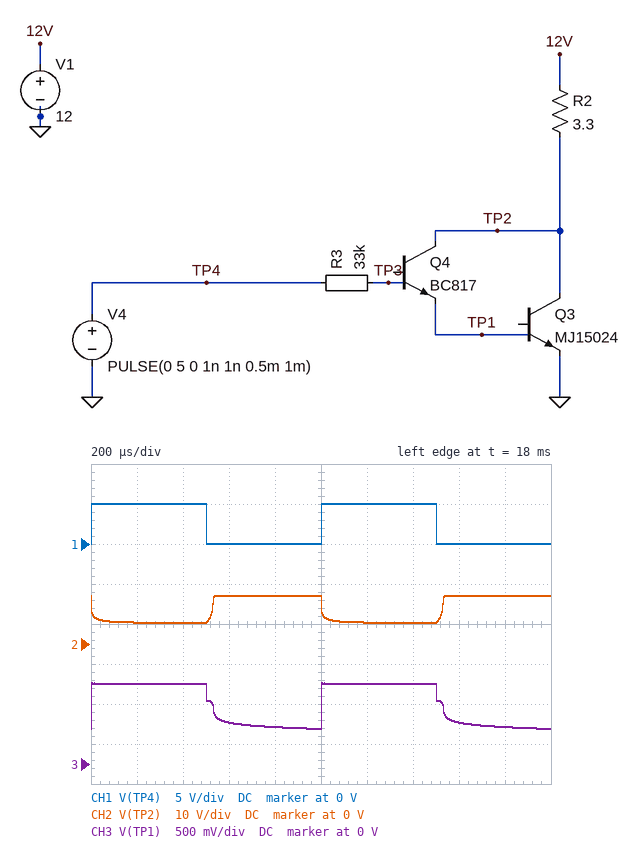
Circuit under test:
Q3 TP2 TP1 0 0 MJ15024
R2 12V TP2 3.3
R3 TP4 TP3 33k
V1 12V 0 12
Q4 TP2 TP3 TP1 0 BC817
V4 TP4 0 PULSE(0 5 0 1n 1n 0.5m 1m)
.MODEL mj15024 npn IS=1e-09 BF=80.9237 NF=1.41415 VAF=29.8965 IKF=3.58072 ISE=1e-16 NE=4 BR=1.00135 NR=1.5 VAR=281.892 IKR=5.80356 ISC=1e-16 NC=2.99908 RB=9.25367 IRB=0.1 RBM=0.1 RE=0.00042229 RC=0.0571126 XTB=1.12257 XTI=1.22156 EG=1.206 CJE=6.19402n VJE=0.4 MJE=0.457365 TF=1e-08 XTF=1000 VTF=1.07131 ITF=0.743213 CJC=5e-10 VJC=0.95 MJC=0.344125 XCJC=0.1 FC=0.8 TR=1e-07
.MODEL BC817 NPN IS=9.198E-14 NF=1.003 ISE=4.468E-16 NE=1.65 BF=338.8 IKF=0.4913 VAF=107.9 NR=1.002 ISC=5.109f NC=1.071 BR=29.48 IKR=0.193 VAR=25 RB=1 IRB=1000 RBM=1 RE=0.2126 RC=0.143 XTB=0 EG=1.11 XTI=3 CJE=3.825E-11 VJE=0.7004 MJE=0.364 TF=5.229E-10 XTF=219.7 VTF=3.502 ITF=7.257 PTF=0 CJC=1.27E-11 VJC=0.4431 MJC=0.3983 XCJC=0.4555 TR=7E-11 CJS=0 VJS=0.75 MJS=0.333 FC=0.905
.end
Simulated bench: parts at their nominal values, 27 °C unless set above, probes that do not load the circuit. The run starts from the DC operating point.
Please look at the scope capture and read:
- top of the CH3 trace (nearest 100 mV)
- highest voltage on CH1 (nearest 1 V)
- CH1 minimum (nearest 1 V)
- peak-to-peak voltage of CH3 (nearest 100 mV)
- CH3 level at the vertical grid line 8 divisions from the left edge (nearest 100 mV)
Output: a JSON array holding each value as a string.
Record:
["1.0 V", "5 V", "0 V", "600 mV", "500 mV"]
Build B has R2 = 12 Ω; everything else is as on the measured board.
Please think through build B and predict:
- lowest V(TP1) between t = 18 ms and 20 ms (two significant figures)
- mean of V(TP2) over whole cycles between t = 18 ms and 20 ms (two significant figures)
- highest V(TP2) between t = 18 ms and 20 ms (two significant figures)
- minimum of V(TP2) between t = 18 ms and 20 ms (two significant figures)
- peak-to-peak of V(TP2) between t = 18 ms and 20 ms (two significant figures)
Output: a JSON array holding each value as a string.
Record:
["470 mV", "4.1 V", "12 V", "940 mV", "11 V"]
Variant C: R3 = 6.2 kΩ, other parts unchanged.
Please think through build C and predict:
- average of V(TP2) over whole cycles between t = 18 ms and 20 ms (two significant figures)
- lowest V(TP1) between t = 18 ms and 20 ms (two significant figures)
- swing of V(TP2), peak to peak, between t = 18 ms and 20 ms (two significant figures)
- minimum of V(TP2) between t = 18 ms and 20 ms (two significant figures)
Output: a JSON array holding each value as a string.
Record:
["3.8 V", "490 mV", "11 V", "1.3 V"]
